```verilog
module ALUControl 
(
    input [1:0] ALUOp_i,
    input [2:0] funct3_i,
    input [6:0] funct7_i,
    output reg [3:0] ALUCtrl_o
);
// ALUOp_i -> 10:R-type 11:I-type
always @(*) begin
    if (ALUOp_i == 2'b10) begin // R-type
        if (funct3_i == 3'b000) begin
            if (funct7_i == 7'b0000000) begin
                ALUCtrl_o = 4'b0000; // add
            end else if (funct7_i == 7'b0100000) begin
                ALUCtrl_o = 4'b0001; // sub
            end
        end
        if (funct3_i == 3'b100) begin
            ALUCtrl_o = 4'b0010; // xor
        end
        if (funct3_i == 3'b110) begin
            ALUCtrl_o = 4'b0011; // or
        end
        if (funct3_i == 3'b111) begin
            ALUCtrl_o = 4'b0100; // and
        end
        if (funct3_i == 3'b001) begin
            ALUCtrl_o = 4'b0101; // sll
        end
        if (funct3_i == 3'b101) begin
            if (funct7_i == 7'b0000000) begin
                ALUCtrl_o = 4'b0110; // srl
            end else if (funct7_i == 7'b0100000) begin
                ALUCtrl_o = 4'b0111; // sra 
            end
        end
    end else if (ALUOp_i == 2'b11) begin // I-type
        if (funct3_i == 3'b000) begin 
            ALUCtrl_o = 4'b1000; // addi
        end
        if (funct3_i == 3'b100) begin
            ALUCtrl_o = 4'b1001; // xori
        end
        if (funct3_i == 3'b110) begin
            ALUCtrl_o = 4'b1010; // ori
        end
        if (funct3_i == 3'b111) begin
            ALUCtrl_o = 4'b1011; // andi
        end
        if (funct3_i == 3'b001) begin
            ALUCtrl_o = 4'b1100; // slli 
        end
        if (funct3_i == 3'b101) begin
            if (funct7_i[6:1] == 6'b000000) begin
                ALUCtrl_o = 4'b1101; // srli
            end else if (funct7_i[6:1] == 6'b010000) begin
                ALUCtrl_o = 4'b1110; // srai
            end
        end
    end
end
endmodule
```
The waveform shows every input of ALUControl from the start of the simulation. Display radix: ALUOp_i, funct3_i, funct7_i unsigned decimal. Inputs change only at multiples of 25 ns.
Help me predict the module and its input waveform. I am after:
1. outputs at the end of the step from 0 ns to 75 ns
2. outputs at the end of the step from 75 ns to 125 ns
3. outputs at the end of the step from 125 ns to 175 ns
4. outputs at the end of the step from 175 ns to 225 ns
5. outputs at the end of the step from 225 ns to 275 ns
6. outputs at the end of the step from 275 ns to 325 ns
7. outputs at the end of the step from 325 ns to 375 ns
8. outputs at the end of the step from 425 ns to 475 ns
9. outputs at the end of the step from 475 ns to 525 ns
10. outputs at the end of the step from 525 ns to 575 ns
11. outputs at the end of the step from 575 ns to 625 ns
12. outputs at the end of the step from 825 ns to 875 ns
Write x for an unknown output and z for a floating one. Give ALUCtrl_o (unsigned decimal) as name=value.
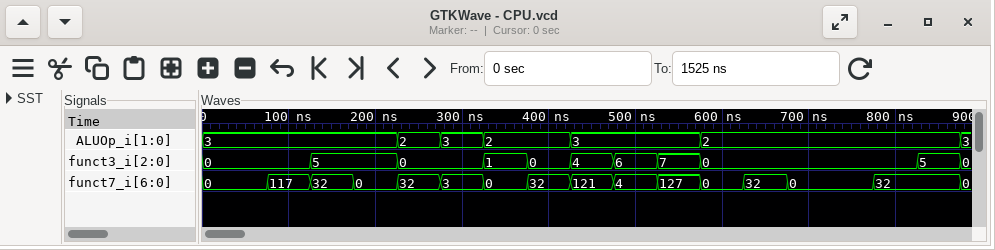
ALUCtrl_o=8
ALUCtrl_o=8
ALUCtrl_o=14
ALUCtrl_o=13
ALUCtrl_o=1
ALUCtrl_o=8
ALUCtrl_o=5
ALUCtrl_o=9
ALUCtrl_o=10
ALUCtrl_o=11
ALUCtrl_o=0
ALUCtrl_o=7
